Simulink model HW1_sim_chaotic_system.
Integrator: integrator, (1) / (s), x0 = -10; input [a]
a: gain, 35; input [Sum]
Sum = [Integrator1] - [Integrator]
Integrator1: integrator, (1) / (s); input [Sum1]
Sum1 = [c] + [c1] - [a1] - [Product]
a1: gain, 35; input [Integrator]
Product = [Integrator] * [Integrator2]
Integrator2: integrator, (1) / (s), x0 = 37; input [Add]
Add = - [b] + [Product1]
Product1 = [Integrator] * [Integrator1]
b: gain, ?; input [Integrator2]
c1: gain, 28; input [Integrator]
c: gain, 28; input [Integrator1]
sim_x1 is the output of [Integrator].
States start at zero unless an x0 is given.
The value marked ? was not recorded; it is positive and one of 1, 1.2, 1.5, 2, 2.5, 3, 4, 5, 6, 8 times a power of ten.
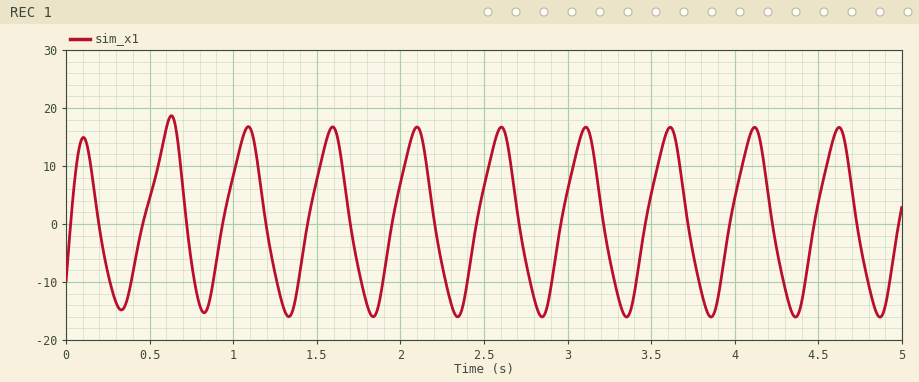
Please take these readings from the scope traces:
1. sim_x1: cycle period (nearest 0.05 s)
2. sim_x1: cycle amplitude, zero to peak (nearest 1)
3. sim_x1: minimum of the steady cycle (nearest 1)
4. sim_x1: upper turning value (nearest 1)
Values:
0.50 s
16
-16
17
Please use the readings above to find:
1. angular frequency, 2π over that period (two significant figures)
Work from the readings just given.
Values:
13 rad/s
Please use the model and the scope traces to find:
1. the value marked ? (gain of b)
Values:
5
